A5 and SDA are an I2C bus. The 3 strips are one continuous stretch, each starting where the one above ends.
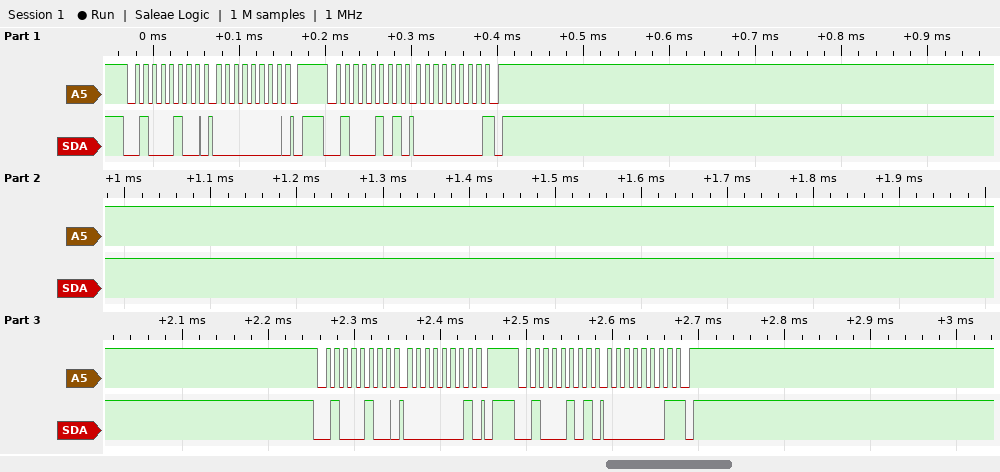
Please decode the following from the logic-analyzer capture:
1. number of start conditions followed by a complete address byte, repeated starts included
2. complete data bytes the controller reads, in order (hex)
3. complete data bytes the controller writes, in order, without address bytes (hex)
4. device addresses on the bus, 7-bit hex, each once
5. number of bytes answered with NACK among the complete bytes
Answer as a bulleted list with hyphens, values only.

- 4
- 00 01
- 00 01
- 0x22
- 2
